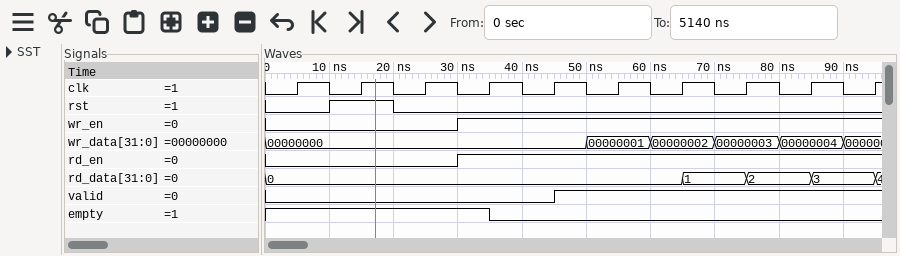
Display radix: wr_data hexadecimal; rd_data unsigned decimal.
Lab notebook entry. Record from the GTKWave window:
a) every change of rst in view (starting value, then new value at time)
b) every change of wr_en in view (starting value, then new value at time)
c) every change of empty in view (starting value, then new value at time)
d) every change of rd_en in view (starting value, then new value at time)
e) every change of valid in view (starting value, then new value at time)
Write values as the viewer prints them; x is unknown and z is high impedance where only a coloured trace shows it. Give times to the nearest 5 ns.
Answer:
0, 1 at 10 ns, 0 at 20 ns
0, 1 at 30 ns
1, 0 at 35 ns
0, 1 at 30 ns
0, 1 at 45 ns
